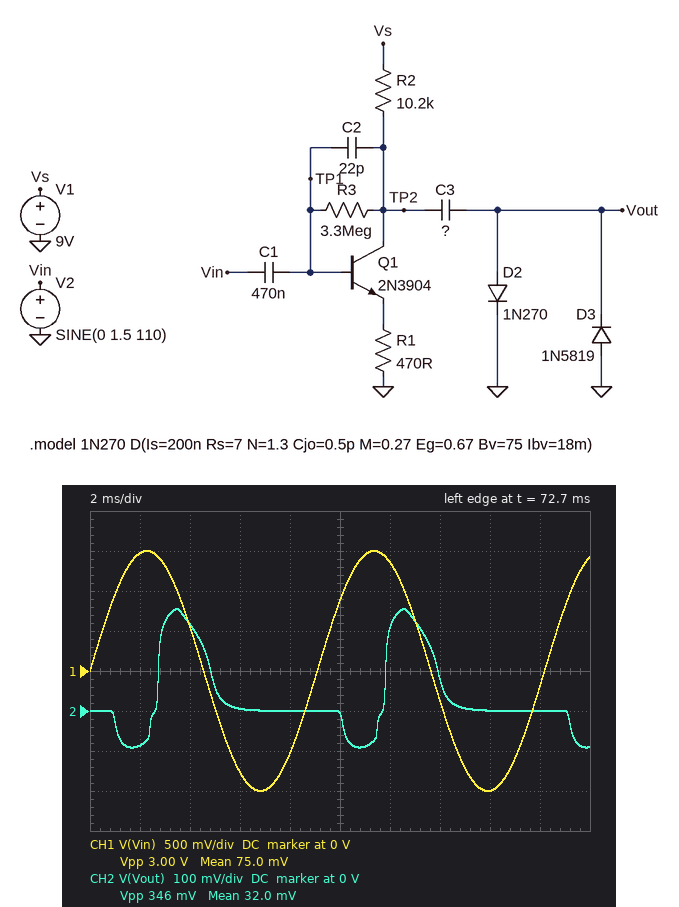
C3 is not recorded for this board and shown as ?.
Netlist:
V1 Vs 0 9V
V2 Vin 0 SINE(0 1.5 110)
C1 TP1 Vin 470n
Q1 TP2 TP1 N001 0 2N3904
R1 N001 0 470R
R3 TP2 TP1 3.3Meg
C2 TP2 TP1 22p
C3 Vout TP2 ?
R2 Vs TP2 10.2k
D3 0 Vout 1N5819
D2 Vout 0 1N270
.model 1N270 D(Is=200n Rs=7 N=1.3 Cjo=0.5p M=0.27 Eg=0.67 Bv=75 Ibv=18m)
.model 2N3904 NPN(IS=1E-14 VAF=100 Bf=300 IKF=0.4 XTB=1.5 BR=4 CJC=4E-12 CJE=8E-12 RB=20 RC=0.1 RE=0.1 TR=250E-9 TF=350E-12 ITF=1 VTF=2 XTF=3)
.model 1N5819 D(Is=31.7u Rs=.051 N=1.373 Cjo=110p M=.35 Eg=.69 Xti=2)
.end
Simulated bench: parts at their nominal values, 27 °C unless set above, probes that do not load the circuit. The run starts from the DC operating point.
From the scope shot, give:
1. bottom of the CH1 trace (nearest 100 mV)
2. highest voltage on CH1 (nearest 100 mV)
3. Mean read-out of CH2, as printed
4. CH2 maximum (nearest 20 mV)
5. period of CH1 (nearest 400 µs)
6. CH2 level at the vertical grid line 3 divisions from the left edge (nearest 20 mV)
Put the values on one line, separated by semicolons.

-1.5 V; 1.5 V; 32.0 mV; 260 mV; 9.2 ms; 0 V
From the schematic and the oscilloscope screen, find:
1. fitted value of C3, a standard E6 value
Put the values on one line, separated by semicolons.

47 nF
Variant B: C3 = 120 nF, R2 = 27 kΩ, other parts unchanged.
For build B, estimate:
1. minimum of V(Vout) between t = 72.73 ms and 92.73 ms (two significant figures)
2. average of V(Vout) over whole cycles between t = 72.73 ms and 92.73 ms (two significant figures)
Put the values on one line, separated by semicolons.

-110 mV; 130 mV
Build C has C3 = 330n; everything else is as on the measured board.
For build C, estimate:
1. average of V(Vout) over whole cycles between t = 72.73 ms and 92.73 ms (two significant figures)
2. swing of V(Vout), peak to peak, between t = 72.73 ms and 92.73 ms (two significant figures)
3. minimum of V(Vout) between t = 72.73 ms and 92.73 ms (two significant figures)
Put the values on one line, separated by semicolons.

140 mV; 390 mV; -120 mV
